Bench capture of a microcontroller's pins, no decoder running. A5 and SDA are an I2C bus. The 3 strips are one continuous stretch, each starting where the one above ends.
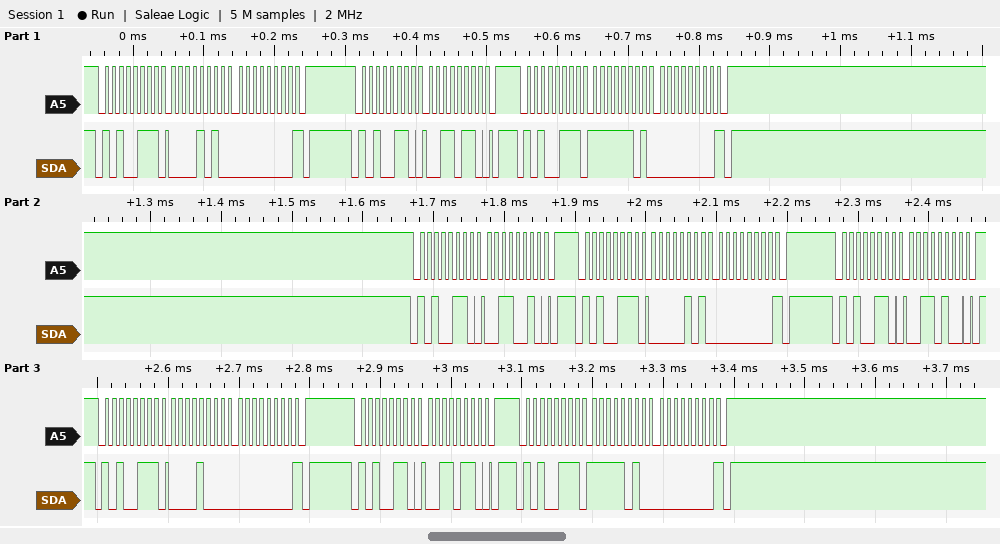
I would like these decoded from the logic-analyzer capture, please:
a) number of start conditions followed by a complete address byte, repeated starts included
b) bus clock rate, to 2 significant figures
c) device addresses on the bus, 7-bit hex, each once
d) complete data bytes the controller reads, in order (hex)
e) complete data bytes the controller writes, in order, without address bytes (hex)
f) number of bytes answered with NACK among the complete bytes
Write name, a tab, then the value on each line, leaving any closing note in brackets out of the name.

number of start conditions followed by a complete address byte, repeated starts included	9
bus clock rate, to 2 significant figures	100 kHz
device addresses on the bus, 7-bit hex, each once	0x53
complete data bytes the controller reads, in order	0A 00 FD 00 05 00 08 00 FA 00
complete data bytes the controller writes, in order, without address bytes	36 32 34 36
number of bytes answered with NACK among the complete bytes	5
